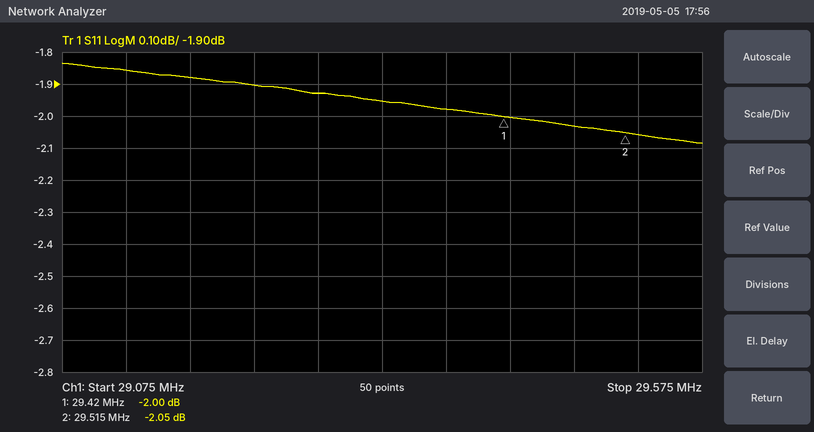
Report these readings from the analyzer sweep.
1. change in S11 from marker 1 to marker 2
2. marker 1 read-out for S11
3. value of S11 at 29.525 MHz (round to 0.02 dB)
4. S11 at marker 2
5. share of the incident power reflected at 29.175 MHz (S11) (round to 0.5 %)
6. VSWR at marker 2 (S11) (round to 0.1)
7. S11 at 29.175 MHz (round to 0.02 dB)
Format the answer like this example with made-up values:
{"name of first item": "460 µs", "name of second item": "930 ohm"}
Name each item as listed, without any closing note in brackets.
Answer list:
{"change in S11 from marker 1 to marker 2": "-0.05 dB", "marker 1 read-out for S11": "-2.00 dB", "value of S11 at 29.525 MHz": "-2.06 dB", "S11 at marker 2": "-2.05 dB", "share of the incident power reflected at 29.175 MHz (S11)": "65.0 %", "VSWR at marker 2 (S11)": "8.5", "S11 at 29.175 MHz": "-1.88 dB"}
